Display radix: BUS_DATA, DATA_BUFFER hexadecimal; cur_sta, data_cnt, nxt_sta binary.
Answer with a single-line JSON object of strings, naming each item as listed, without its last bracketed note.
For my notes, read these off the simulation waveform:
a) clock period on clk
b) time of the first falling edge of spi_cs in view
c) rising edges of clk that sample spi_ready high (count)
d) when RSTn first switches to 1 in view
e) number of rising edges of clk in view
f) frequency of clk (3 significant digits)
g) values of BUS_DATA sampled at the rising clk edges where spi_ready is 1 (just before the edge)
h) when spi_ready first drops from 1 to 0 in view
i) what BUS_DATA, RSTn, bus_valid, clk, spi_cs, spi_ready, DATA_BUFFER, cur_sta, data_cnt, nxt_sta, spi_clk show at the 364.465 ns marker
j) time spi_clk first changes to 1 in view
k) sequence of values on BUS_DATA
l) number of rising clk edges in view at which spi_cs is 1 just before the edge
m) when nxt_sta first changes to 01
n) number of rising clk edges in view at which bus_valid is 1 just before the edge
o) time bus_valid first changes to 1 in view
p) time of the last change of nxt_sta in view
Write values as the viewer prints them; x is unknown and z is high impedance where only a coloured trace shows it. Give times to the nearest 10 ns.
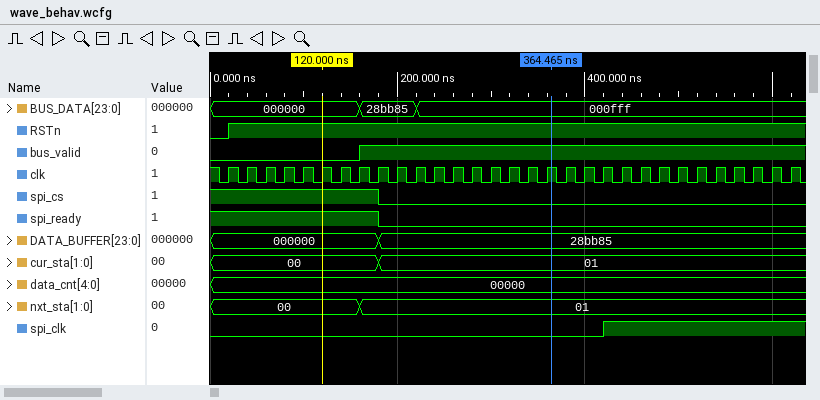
{"clock period on clk": "20 ns", "time of the first falling edge of spi_cs in view": "180 ns", "rising edges of clk that sample spi_ready high": "9", "when RSTn first switches to 1 in view": "20 ns", "number of rising edges of clk in view": "31", "frequency of clk": "50.0 MHz", "values of BUS_DATA sampled at the rising clk edges where spi_ready is 1": "000000, 000000, 000000, 000000, 000000, 000000, 000000, 000000, 28bb85", "when spi_ready first drops from 1 to 0 in view": "180 ns", "what BUS_DATA, RSTn, bus_valid, clk, spi_cs, spi_ready, DATA_BUFFER, cur_sta, data_cnt, nxt_sta, spi_clk show at the 364.465 ns marker": "BUS_DATA=000fff, RSTn=1, bus_valid=1, clk=1, spi_cs=0, spi_ready=0, DATA_BUFFER=28bb85, cur_sta=01, data_cnt=00000, nxt_sta=01, spi_clk=0", "time spi_clk first changes to 1 in view": "420 ns", "sequence of values on BUS_DATA": "000000, 28bb85, 000fff", "number of rising clk edges in view at which spi_cs is 1 just before the edge": "9", "when nxt_sta first changes to 01": "160 ns", "number of rising clk edges in view at which bus_valid is 1 just before the edge": "23", "time bus_valid first changes to 1 in view": "160 ns", "time of the last change of nxt_sta in view": "160 ns"}
